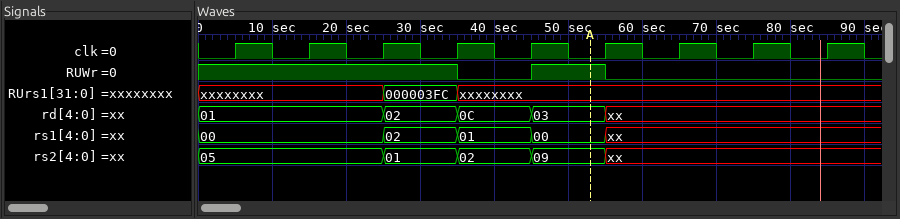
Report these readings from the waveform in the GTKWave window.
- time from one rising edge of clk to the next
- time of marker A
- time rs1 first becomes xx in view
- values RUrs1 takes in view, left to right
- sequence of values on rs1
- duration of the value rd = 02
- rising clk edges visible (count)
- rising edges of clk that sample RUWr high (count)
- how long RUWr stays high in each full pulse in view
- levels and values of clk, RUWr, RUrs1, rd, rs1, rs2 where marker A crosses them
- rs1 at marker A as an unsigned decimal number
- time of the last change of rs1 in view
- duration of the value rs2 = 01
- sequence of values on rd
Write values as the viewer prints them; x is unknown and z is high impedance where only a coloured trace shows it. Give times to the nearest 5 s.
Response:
10 s
55 s
55 s
xxxxxxxx, 000003FC, xxxxxxxx
00, 02, 01, 00, xx
10 s
9
5
10 s
clk=0, RUWr=1, RUrs1=xxxxxxxx, rd=03, rs1=00, rs2=09
0
55 s
10 s
01, 02, 0C, 03, xx
